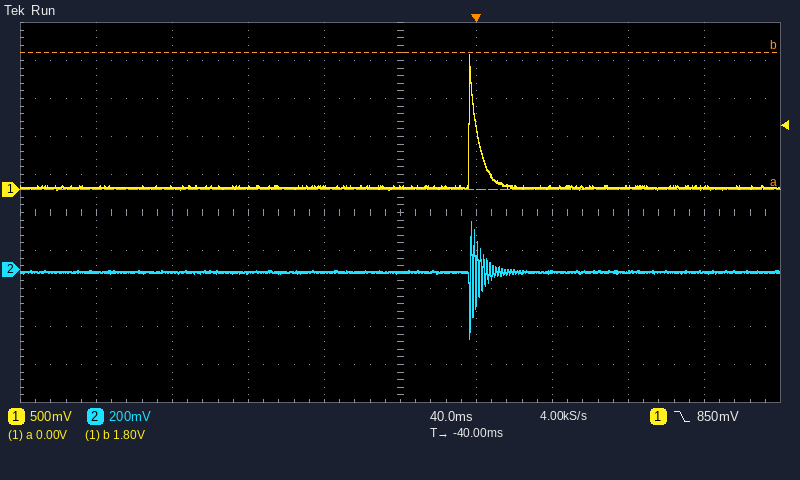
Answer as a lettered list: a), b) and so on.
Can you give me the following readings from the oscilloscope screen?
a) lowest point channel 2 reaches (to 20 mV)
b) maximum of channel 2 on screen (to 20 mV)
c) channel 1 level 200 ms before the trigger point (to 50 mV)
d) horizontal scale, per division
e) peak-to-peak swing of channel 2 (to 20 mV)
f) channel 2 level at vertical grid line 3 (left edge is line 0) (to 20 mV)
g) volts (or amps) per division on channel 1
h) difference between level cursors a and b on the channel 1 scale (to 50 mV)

a) -360 mV
b) 260 mV
c) 50 mV
d) 40 ms
e) 620 mV
f) -20 mV
g) 500 mV
h) 1.80 V
